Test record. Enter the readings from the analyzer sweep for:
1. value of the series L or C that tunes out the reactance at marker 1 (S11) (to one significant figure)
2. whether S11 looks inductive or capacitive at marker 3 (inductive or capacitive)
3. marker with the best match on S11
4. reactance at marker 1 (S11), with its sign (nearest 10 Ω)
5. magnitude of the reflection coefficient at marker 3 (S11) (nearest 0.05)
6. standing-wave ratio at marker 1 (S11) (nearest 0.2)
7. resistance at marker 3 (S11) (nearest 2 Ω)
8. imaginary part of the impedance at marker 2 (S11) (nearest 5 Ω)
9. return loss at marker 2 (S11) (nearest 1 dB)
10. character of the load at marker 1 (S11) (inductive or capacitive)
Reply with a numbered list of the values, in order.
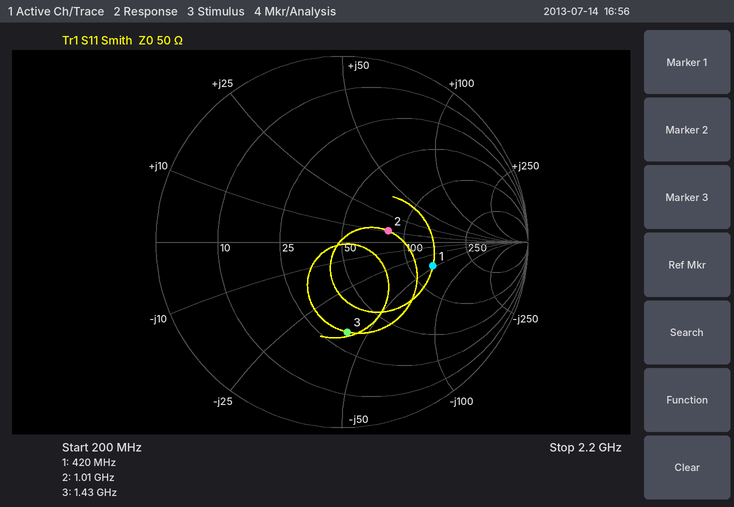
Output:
1. 20 nH
2. capacitive
3. marker 2
4. -50 Ω
5. 0.50
6. 3.0
7. 32 Ω
8. +10 Ω
9. 12 dB
10. capacitive
